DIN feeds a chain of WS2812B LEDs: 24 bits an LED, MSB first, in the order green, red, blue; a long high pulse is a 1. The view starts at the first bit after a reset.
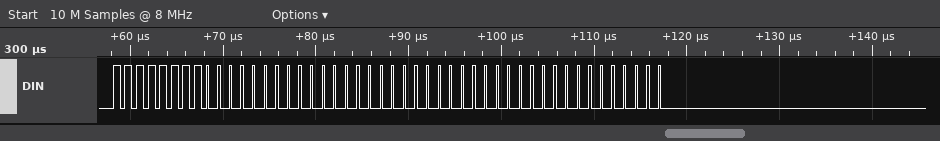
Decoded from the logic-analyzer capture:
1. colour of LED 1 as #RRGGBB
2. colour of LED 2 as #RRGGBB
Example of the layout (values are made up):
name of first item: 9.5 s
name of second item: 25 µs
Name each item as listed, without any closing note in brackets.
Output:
colour of LED 1 as #RRGGBB: #00FF00
colour of LED 2 as #RRGGBB: #000000
